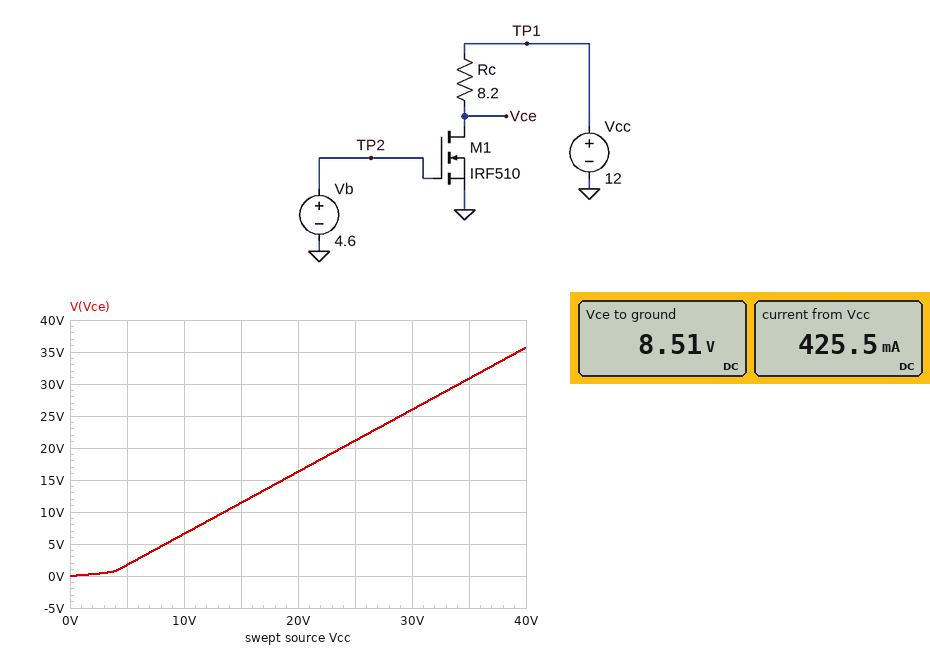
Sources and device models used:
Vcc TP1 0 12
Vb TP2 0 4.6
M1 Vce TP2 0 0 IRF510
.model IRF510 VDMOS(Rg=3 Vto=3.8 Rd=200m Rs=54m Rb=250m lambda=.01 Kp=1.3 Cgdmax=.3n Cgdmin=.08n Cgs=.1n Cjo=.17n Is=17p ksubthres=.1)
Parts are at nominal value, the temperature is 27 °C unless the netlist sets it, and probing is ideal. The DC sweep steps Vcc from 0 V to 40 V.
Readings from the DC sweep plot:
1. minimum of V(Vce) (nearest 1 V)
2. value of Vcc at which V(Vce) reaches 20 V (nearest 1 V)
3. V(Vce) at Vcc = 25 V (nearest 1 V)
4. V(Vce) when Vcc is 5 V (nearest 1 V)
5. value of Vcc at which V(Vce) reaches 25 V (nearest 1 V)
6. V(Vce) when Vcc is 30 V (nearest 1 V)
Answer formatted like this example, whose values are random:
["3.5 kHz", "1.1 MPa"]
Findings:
["0 V", "24 V", "21 V", "2 V", "29 V", "26 V"]
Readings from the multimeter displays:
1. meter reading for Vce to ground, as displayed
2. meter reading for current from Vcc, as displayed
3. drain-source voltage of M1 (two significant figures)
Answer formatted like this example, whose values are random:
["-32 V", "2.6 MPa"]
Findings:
["8.51 V", "425.5 mA", "8.5 V"]
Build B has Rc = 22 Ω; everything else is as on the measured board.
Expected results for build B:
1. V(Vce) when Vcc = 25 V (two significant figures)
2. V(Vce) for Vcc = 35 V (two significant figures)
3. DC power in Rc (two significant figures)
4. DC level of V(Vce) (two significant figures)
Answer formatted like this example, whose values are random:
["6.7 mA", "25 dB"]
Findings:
["15 V", "24 V", "3.6 W", "3.1 V"]
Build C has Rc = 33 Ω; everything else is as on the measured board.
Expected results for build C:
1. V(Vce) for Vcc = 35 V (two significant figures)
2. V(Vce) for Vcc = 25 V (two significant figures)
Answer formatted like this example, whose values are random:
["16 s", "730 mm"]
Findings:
["20 V", "11 V"]
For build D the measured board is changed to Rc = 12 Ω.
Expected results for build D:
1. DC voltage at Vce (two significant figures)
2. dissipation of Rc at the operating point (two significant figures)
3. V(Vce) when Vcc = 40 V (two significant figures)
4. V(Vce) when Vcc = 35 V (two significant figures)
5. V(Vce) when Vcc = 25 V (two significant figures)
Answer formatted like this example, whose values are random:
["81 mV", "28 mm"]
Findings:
["7.0 V", "2.1 W", "34 V", "29 V", "19 V"]
